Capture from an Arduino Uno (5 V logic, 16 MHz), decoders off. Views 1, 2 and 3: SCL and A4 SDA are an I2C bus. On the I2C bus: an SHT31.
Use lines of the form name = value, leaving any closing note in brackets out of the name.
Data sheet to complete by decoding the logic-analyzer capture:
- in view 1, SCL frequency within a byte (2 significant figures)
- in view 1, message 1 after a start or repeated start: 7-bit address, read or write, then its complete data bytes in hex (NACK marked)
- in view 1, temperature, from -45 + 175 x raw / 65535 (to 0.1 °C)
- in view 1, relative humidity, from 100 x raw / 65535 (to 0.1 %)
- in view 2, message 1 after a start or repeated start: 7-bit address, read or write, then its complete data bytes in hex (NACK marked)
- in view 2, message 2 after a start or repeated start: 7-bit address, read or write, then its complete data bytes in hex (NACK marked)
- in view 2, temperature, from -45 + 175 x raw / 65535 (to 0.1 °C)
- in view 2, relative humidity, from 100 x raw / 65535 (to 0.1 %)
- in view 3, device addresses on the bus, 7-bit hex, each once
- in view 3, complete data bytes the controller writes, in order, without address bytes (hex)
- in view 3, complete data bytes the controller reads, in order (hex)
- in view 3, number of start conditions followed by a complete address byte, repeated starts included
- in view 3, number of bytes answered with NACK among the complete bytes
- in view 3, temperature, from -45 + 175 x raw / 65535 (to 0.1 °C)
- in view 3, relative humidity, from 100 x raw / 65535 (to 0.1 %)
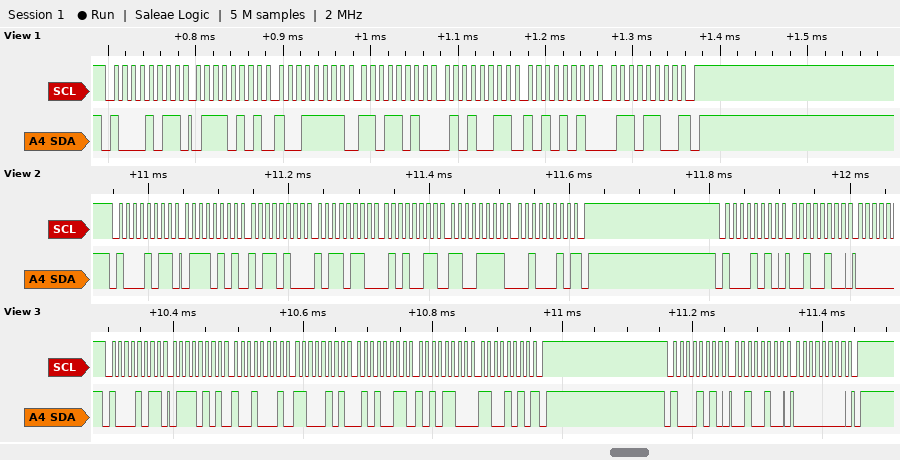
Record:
in view 1, SCL frequency within a byte = 100 kHz
in view 1, message 1 after a start or repeated start: 7-bit address, read or write, then its complete data bytes in hex = 0x45 read: 75 9F DA 53 AA 6C NACK
in view 1, temperature, from -45 + 175 x raw / 65535 = 35.4 °C
in view 1, relative humidity, from 100 x raw / 65535 = 32.7 %
in view 2, message 1 after a start or repeated start: 7-bit address, read or write, then its complete data bytes in hex = 0x45 read: 75 B4 B6 53 CF 22 NACK
in view 2, message 2 after a start or repeated start: 7-bit address, read or write, then its complete data bytes in hex = 0x45 write: 24
in view 2, temperature, from -45 + 175 x raw / 65535 = 35.5 °C
in view 2, relative humidity, from 100 x raw / 65535 = 32.7 %
in view 3, device addresses on the bus, 7-bit hex, each once = 0x45
in view 3, complete data bytes the controller writes, in order, without address bytes = 24 00
in view 3, complete data bytes the controller reads, in order = 75 91 C5 53 AC CA
in view 3, number of start conditions followed by a complete address byte, repeated starts included = 2
in view 3, number of bytes answered with NACK among the complete bytes = 1
in view 3, temperature, from -45 + 175 x raw / 65535 = 35.4 °C
in view 3, relative humidity, from 100 x raw / 65535 = 32.7 %
